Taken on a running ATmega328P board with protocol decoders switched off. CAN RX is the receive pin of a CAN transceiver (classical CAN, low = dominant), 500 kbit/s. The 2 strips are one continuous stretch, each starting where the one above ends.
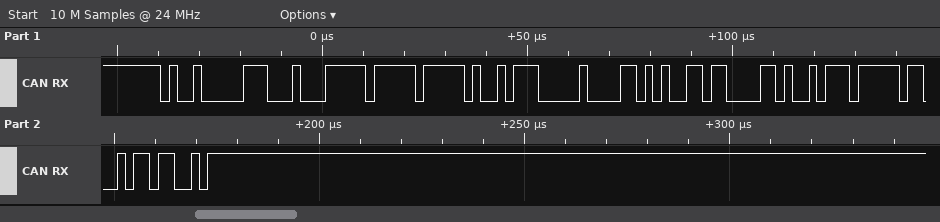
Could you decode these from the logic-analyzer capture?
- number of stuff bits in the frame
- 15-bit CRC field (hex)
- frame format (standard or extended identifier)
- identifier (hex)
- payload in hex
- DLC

6
0x796C
standard
0x483
FF FF 2E 00 D4 D8 69 77
8
